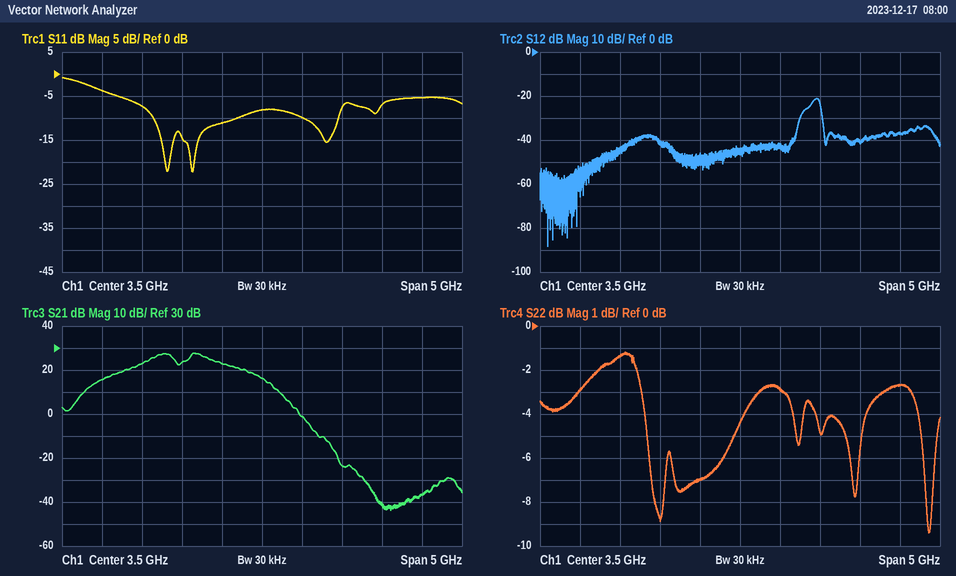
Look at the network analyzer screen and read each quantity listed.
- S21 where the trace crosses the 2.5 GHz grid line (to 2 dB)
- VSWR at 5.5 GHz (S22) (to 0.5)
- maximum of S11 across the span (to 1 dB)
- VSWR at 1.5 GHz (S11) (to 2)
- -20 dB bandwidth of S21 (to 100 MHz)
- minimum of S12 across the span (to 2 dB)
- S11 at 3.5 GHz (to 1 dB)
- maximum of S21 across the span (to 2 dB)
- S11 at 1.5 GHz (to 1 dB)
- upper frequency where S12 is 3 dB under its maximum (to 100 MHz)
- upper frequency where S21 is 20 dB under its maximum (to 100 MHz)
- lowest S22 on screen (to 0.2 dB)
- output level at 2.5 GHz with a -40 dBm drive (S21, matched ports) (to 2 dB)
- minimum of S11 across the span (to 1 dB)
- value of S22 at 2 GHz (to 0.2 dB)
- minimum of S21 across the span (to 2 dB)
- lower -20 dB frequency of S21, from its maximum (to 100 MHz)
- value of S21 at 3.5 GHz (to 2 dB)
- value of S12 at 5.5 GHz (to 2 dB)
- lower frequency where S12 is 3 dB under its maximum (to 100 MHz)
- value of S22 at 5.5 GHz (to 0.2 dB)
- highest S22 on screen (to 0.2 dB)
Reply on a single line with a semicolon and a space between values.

24 dB; 6.5; -1 dB; 4; 2.6 GHz; -88 dB; -8 dB; 28 dB; -4 dB; 4.5 GHz; 3.8 GHz; -9.4 dB; -16 dBm; -22 dB; -1.4 dB; -44 dB; 1.2 GHz; 16 dB; -36 dB; 4.4 GHz; -2.6 dB; -1.2 dB
